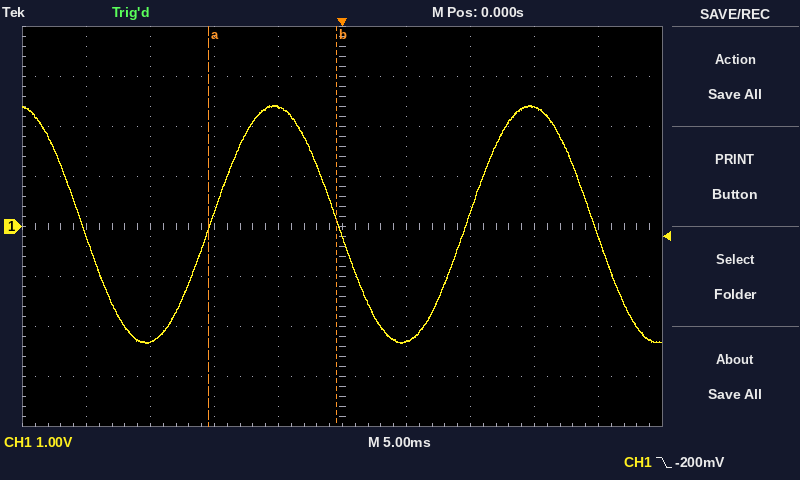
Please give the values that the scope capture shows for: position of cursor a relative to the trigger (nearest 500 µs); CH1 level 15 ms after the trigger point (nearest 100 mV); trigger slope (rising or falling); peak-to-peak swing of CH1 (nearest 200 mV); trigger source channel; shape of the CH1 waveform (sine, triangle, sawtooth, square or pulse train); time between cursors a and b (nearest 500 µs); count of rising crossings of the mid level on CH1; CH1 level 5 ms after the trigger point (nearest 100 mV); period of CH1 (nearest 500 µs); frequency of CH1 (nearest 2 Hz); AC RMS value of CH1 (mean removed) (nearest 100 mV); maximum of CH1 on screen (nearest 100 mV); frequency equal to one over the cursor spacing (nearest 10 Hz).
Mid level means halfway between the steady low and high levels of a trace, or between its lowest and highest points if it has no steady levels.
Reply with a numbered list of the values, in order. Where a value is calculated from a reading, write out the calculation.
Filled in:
1. -10.5 ms
2. 2.4 V
3. falling
4. 4.8 V
5. CH1
6. sine
7. 10.0 ms
8. 2
9. -2.3 V
10. 20.0 ms
11. 1 / 20.0 ms ≈ 50 Hz
12. 4.8 V / (2√2) ≈ 1.7 V
13. 2.4 V
14. 1 / 10.0 ms ≈ 100 Hz
